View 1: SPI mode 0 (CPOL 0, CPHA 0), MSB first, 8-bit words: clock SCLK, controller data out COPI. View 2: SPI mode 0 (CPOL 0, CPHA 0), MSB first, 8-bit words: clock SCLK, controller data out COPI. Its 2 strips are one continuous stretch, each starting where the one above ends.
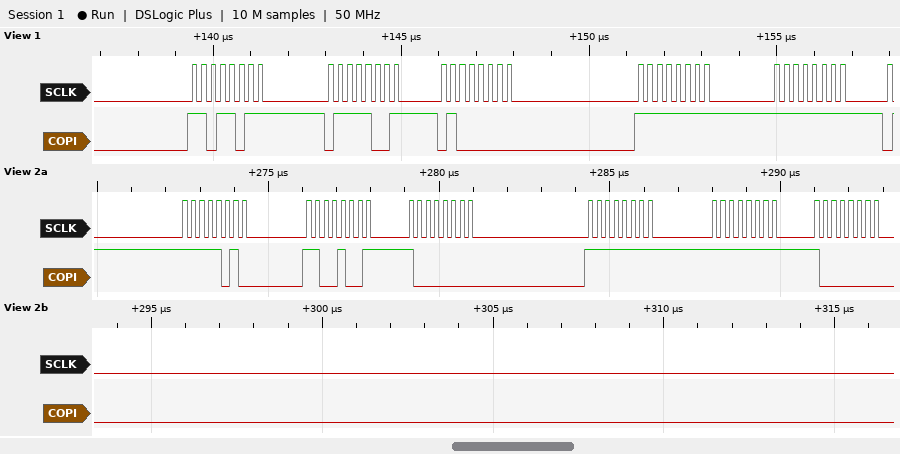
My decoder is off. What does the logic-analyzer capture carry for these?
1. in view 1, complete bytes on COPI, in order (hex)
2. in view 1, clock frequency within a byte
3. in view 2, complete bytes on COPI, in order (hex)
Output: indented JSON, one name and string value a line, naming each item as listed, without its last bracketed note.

{
  "in view 1, complete bytes on COPI, in order": "0xDB 0x79 0x40 0xFF 0xFF",
  "in view 1, clock frequency within a byte": "4 MHz",
  "in view 2, complete bytes on COPI, in order": "0xFA 0xC9 0x80 0xFF 0xFF 0x80"
}
